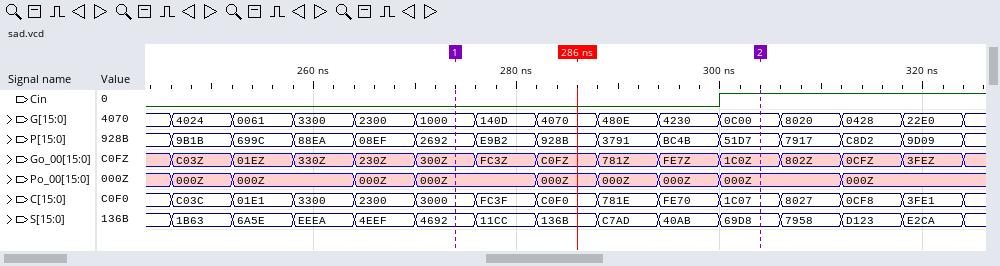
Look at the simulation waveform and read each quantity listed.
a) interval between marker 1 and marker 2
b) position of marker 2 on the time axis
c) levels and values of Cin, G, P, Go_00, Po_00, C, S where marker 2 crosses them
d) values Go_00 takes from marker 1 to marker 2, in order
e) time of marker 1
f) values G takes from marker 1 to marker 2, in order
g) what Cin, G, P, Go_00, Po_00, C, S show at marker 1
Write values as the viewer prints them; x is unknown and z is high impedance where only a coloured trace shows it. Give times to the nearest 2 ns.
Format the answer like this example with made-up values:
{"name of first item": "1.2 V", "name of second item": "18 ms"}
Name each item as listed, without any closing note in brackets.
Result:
{"interval between marker 1 and marker 2": "30 ns", "position of marker 2 on the time axis": "304 ns", "levels and values of Cin, G, P, Go_00, Po_00, C, S where marker 2 crosses them": "Cin=1, G=0C00, P=51D7, Go_00=1C0Z, Po_00=000Z, C=1C07, S=69D8", "values Go_00 takes from marker 1 to marker 2, in order": "300Z, FC3Z, C0FZ, 781Z, FE7Z, 1C0Z", "time of marker 1": "274 ns", "values G takes from marker 1 to marker 2, in order": "1000, 140D, 4070, 480E, 4230, 0C00", "what Cin, G, P, Go_00, Po_00, C, S show at marker 1": "Cin=0, G=1000, P=2692, Go_00=300Z, Po_00=000Z, C=3000, S=4692"}
